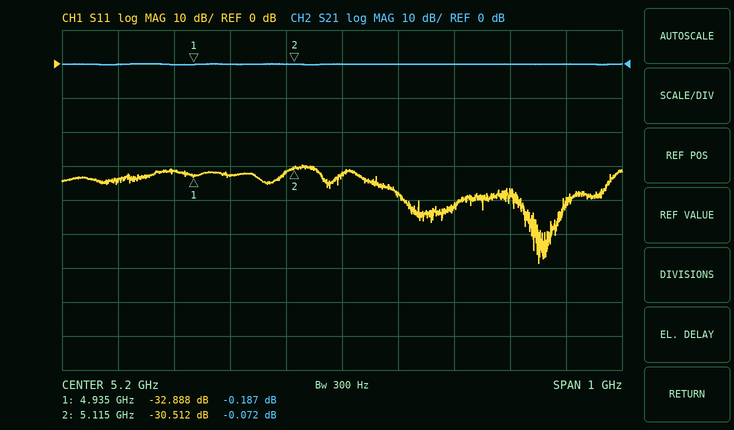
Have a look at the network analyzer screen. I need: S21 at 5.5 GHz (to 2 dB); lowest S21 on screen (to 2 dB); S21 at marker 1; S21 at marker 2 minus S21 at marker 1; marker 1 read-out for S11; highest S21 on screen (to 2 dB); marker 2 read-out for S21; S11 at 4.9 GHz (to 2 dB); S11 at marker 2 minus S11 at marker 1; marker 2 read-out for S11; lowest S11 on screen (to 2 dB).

0 dB
0 dB
-0.187 dB
0.115 dB
-32.888 dB
0 dB
-0.072 dB
-32 dB
2.376 dB
-30.512 dB
-58 dB
